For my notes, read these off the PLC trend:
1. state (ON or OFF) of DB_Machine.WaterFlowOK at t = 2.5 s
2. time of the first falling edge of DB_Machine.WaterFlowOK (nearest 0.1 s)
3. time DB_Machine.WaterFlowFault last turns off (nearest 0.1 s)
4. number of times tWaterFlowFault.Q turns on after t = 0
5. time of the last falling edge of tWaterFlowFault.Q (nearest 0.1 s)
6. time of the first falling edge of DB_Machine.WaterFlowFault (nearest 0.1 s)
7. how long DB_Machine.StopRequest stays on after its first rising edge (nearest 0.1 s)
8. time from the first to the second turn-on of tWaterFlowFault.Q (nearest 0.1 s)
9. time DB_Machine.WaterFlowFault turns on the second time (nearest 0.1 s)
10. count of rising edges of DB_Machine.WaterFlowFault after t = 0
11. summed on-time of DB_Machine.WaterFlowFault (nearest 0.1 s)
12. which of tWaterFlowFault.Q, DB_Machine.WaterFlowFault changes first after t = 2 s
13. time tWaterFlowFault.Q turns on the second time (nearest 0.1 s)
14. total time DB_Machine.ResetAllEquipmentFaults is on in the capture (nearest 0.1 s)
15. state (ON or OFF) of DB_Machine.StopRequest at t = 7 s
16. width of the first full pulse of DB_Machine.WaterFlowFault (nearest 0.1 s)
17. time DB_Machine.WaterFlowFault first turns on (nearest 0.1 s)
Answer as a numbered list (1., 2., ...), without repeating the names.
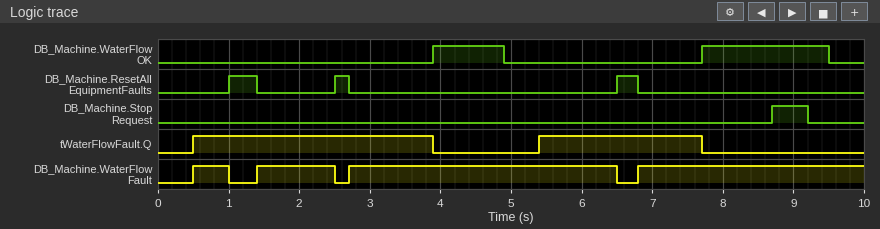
1. OFF
2. 4.9 s
3. 6.5 s
4. 2
5. 7.7 s
6. 1.0 s
7. 0.5 s
8. 4.9 s
9. 1.4 s
10. 4
11. 8.6 s
12. DB_Machine.WaterFlowFault
13. 5.4 s
14. 0.9 s
15. OFF
16. 0.5 s
17. 0.5 s
